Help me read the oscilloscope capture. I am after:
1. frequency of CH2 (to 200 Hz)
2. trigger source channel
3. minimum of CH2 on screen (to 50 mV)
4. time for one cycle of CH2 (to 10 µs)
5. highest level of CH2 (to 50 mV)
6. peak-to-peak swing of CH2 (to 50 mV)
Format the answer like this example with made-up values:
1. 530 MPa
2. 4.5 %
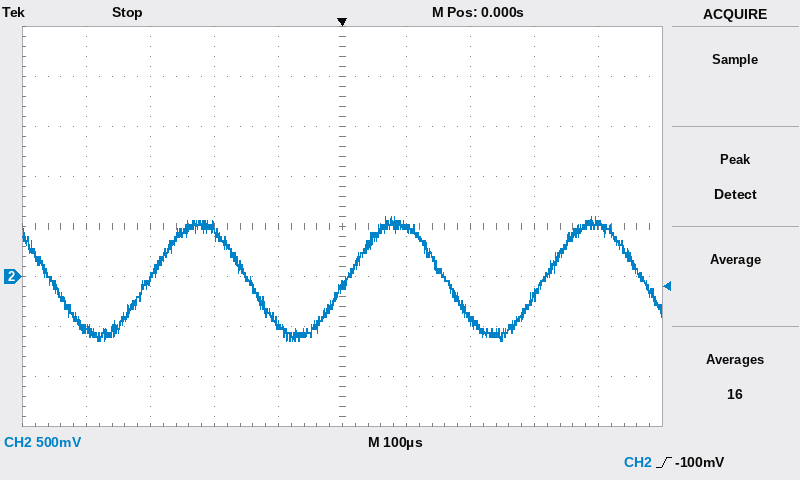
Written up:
1. 3.2 kHz
2. CH2
3. -650 mV
4. 310 µs
5. 600 mV
6. 1.25 V
